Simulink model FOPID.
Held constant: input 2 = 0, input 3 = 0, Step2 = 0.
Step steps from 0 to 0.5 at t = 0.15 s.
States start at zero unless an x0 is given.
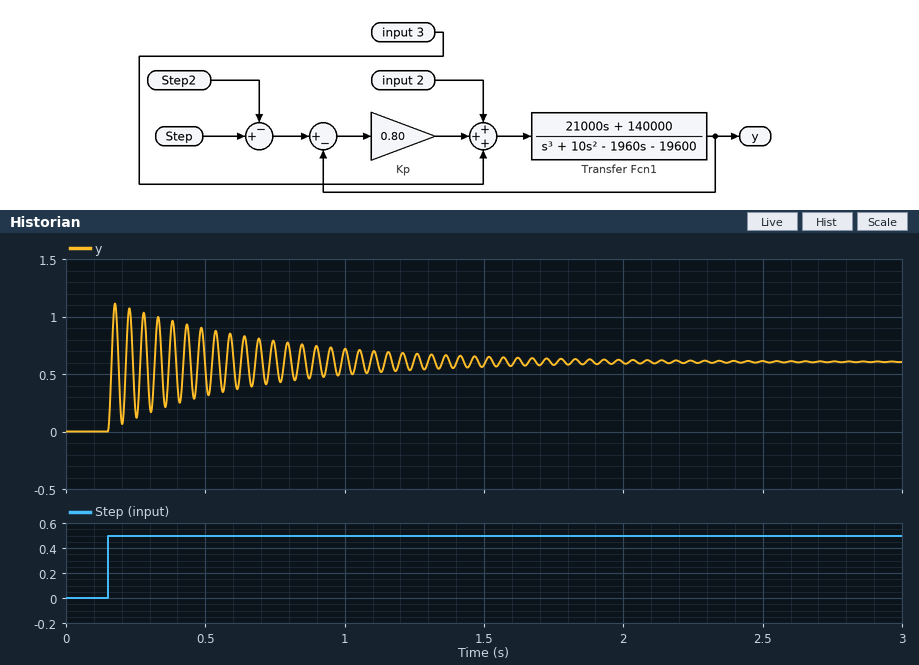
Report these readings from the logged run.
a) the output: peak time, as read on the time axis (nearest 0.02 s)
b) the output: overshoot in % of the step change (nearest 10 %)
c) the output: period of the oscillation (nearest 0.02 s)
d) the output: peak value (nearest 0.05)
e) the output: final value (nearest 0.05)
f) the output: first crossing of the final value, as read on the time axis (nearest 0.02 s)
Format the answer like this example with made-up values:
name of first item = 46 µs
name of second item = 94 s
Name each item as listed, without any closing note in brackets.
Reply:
the output: peak time, as read on the time axis = 0.18 s
the output: overshoot in % of the step change = 80 %
the output: period of the oscillation = 0.06 s
the output: peak value = 1.10
the output: final value = 0.60
the output: first crossing of the final value, as read on the time axis = 0.16 s
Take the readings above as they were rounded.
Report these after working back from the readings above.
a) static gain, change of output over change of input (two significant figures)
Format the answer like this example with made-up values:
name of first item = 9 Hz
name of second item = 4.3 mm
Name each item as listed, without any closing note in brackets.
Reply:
static gain, change of output over change of input = 1.2
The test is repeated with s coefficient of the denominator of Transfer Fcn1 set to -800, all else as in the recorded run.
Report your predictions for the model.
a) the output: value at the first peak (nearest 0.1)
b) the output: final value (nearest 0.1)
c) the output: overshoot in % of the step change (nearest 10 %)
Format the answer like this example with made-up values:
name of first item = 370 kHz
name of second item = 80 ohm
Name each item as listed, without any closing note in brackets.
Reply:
the output: value at the first peak = 1.0
the output: final value = 0.6
the output: overshoot in % of the step change = 70 %
